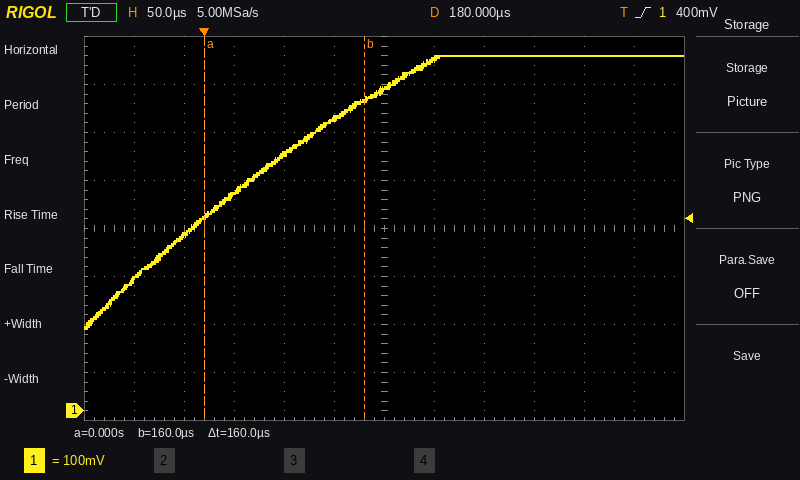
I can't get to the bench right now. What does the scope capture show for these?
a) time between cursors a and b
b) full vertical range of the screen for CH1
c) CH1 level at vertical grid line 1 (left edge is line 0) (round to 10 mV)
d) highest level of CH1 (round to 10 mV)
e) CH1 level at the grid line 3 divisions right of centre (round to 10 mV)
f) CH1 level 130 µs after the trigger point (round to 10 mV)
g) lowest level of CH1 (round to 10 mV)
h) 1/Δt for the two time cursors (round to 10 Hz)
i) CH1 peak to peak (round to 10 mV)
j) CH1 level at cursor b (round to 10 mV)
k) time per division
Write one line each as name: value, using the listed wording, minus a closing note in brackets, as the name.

time between cursors a and b: 160 µs
full vertical range of the screen for CH1: 800 mV
CH1 level at vertical grid line 1 (left edge is line 0): 270 mV
highest level of CH1: 740 mV
CH1 level at the grid line 3 divisions right of centre: 740 mV
CH1 level 130 µs after the trigger point: 610 mV
lowest level of CH1: 170 mV
1/Δt for the two time cursors: 6.25 kHz
CH1 peak to peak: 570 mV
CH1 level at cursor b: 650 mV
time per division: 50 µs
